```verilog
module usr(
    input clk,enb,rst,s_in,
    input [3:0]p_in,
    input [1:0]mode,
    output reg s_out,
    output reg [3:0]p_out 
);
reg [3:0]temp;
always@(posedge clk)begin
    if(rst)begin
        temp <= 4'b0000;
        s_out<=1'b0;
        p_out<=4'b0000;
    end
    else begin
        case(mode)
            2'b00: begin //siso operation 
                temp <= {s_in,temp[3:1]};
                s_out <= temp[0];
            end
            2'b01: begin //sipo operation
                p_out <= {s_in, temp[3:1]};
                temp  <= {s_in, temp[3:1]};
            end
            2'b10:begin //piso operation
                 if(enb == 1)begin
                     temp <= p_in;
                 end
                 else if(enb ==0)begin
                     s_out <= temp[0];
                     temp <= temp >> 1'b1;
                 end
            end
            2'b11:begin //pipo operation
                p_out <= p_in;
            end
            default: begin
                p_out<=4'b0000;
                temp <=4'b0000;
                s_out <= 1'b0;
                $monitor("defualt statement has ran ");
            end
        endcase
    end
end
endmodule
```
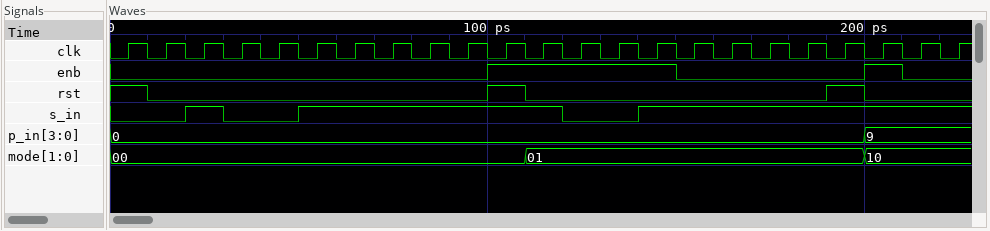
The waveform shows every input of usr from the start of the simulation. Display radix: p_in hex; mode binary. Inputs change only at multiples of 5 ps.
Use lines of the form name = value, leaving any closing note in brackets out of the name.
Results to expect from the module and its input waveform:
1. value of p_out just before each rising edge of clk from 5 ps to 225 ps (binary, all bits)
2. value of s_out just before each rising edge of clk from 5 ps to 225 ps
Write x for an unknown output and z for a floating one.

value of p_out just before each rising edge of clk from 5 ps to 225 ps = x, 0000, 0000, 0000, 0000, 0000, 0000, 0000, 0000, 0000, 0000, 0000, 1000, 0100, 0010, 1001, 1100, 1110, 1111, 1111, 0000, 0000, 0000
value of s_out just before each rising edge of clk from 5 ps to 225 ps = x 0 0 0 0 0 0 1 0 0 1 0 0 0 0 0 0 0 0 0 0 0 1
